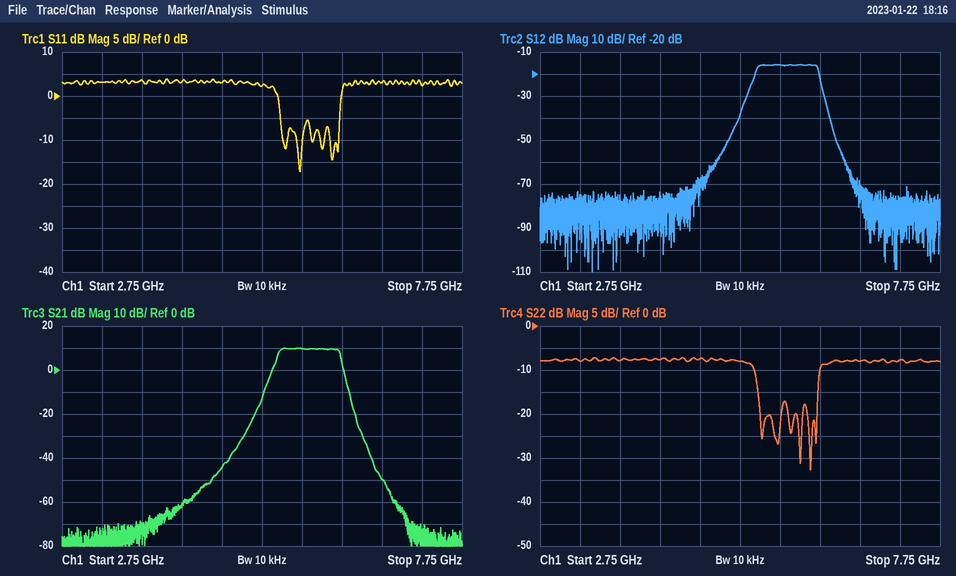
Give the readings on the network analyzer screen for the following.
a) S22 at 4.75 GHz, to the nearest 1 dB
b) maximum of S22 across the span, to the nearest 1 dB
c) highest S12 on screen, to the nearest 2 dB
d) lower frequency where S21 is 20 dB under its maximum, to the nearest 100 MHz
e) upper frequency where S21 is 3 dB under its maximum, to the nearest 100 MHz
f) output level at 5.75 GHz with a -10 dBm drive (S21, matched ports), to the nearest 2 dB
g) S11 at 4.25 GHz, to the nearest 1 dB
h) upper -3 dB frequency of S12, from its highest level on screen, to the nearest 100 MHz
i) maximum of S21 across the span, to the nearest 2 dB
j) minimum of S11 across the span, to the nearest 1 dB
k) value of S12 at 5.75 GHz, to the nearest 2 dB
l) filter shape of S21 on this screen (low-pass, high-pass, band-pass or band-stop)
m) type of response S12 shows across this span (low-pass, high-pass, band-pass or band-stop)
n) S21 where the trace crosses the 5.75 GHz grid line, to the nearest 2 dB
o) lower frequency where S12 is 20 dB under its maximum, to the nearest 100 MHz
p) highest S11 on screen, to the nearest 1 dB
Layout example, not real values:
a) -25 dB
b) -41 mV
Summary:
a) -7 dB
b) -7 dB
c) -16 dB
d) 5.3 GHz
e) 6.2 GHz
f) 0 dBm
g) 3 dB
h) 6.2 GHz
i) 10 dB
j) -17 dB
k) -16 dB
l) band-pass
m) band-pass
n) 10 dB
o) 5.3 GHz
p) 4 dB
